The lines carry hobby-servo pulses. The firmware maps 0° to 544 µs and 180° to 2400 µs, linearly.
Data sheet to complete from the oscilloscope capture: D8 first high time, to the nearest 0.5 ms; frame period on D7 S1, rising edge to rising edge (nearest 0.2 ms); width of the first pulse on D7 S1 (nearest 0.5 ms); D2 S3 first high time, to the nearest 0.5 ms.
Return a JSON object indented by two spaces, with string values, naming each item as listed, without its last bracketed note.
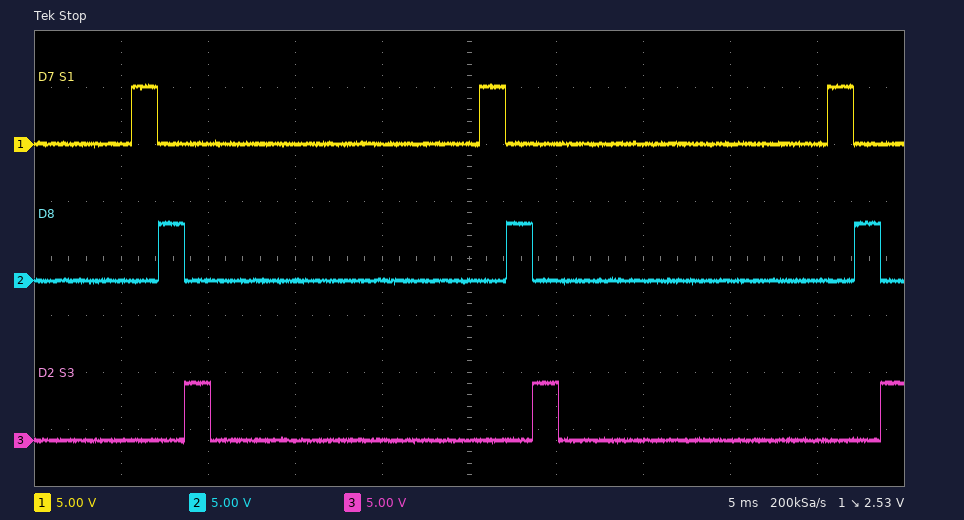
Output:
{
  "D8 first high time, to the nearest 0.5 ms": "1.5 ms",
  "frame period on D7 S1, rising edge to rising edge": "20.0 ms",
  "width of the first pulse on D7 S1": "1.5 ms",
  "D2 S3 first high time, to the nearest 0.5 ms": "1.5 ms"
}
